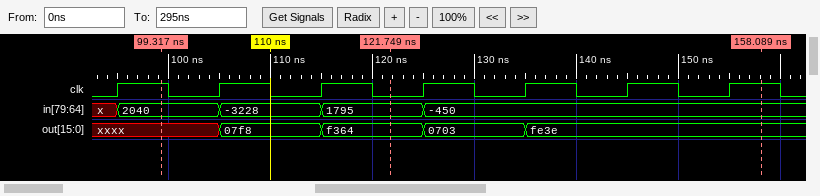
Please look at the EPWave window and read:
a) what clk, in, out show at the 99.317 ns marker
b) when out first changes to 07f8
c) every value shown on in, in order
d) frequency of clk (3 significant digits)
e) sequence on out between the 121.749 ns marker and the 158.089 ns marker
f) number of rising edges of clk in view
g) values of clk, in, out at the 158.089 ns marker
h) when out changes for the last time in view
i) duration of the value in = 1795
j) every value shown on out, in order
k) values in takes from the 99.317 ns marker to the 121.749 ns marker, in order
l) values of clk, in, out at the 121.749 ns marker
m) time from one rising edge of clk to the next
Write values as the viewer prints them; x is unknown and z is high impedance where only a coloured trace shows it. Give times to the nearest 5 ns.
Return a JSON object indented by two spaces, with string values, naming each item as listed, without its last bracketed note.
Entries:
{
  "what clk, in, out show at the 99.317 ns marker": "clk=1, in=2040, out=xxxx",
  "when out first changes to 07f8": "105 ns",
  "every value shown on in, in order": "x, 2040, -3228, 1795, -450",
  "frequency of clk": "100 MHz",
  "sequence on out between the 121.749 ns marker and the 158.089 ns marker": "f364, 0703, fe3e",
  "number of rising edges of clk in view": "7",
  "values of clk, in, out at the 158.089 ns marker": "clk=1, in=-450, out=fe3e",
  "when out changes for the last time in view": "135 ns",
  "duration of the value in = 1795": "10 ns",
  "every value shown on out, in order": "xxxx, 07f8, f364, 0703, fe3e",
  "values in takes from the 99.317 ns marker to the 121.749 ns marker, in order": "2040, -3228, 1795",
  "values of clk, in, out at the 121.749 ns marker": "clk=0, in=1795, out=f364",
  "time from one rising edge of clk to the next": "10 ns"
}
